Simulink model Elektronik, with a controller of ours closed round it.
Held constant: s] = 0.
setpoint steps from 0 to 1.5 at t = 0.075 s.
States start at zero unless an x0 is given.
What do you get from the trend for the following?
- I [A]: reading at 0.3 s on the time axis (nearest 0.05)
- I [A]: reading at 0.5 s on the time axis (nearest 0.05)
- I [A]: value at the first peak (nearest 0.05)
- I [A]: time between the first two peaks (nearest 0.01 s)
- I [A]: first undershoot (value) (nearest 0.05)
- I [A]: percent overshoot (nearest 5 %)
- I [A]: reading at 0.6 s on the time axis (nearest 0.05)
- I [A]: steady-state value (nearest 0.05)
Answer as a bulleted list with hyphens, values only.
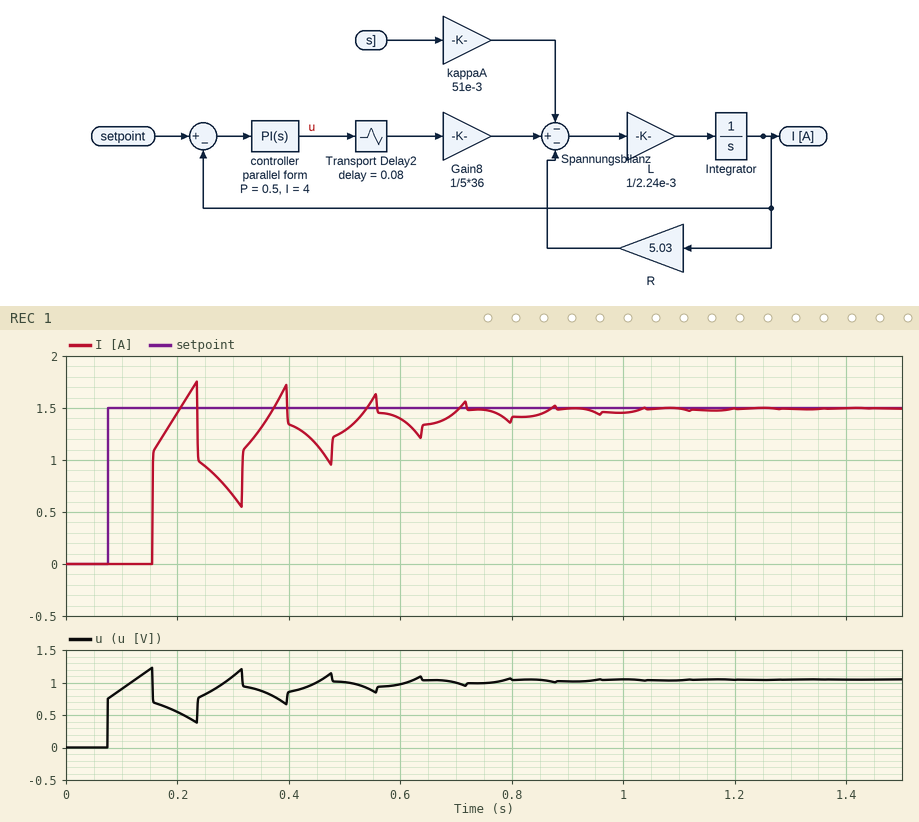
- 0.65
- 1.30
- 1.75
- 0.16 s
- 0.55
- 15 %
- 1.40
- 1.50
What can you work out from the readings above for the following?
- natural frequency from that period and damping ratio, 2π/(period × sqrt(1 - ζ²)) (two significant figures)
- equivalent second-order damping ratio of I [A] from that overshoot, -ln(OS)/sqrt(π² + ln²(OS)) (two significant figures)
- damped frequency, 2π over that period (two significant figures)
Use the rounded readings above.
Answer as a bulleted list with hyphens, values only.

- 46 rad/s
- 0.52
- 39 rad/s
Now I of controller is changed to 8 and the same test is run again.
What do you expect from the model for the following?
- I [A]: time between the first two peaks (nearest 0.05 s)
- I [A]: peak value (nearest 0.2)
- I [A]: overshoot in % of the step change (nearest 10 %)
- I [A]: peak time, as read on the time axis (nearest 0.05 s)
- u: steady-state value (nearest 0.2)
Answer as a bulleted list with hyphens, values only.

- 0.15 s
- 2.4
- 60 %
- 0.25 s
- 1.0
